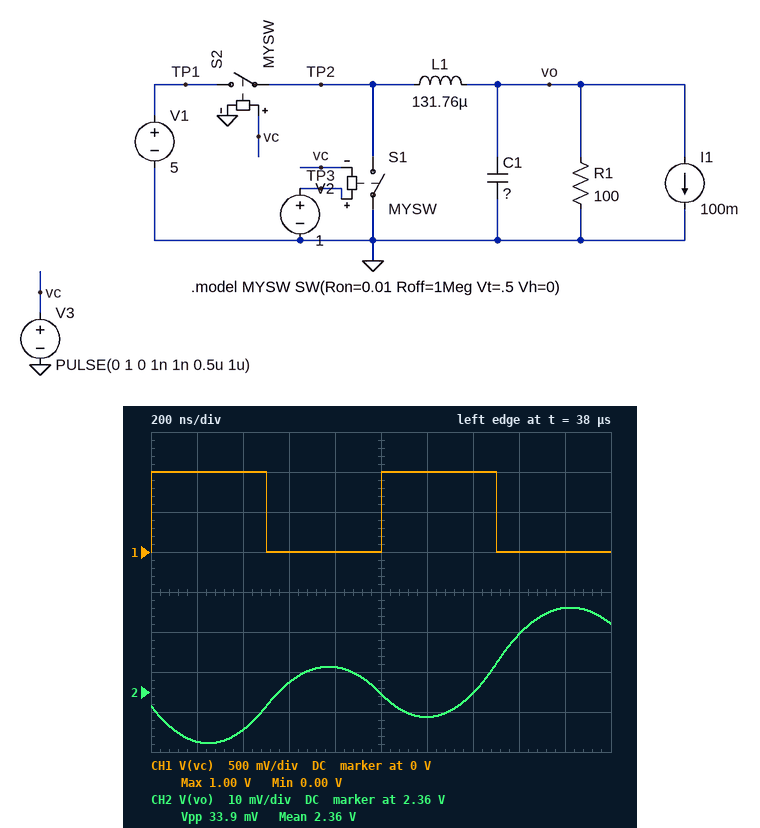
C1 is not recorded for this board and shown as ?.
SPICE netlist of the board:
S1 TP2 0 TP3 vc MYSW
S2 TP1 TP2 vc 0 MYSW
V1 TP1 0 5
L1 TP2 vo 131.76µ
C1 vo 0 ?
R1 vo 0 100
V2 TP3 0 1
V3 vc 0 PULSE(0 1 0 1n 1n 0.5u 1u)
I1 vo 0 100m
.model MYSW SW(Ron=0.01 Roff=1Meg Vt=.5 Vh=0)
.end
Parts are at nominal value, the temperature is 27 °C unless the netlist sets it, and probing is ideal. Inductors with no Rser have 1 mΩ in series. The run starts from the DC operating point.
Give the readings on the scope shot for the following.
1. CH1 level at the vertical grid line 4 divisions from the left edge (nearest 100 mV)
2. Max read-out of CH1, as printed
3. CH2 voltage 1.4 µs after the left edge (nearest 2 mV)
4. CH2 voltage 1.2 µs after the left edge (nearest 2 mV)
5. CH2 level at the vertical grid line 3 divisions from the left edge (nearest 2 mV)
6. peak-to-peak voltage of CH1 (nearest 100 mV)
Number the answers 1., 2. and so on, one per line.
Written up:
1. 0 V
2. 1.00 V
3. 2.360 V
4. 2.354 V
5. 2.362 V
6. 1.0 V
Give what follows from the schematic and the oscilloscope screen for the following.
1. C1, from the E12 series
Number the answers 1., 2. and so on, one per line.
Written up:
1. 68 nF
